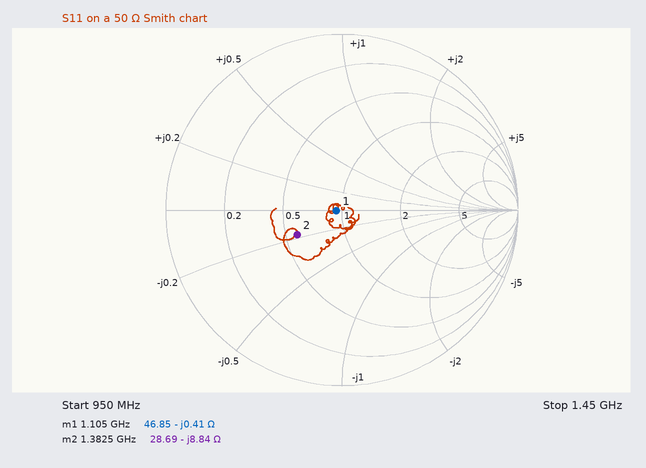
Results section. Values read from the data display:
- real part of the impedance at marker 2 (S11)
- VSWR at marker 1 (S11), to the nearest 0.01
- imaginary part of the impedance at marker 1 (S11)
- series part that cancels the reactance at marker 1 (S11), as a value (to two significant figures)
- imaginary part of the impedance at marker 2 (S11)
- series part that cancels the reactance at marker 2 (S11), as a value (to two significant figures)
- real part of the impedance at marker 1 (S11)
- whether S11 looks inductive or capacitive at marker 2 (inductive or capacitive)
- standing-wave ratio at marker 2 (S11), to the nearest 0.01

28.69 Ω
1.07
-0.41 Ω
59 pH
-8.84 Ω
1.0 nH
46.85 Ω
capacitive
1.82
